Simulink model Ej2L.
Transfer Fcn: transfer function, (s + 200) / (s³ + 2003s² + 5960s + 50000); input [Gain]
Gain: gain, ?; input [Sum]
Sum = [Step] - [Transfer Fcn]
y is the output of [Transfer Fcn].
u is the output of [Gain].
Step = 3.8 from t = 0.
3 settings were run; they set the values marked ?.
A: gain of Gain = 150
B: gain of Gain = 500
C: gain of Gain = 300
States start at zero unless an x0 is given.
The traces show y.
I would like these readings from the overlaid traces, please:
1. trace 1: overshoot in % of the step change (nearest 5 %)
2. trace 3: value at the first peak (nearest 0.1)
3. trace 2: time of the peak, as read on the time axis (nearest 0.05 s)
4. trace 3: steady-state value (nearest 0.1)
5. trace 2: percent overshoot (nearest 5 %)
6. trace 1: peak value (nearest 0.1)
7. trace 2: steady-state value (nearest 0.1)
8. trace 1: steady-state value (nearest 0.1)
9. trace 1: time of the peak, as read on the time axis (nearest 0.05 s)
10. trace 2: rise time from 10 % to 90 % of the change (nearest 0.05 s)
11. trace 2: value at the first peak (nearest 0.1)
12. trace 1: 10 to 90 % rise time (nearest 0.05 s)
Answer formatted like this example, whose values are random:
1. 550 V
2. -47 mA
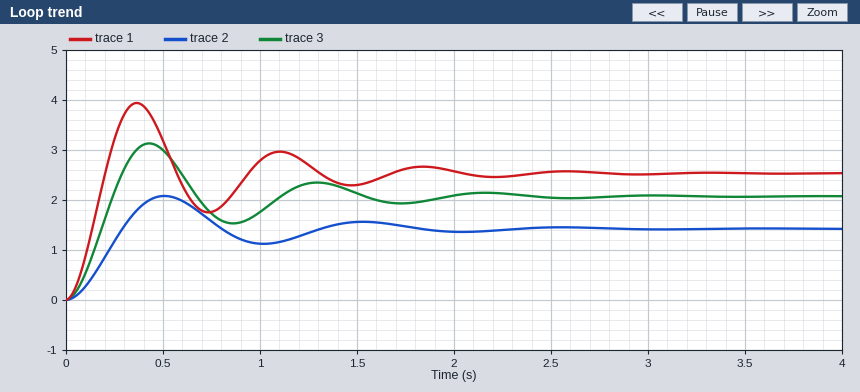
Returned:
1. 55 %
2. 3.1
3. 0.50 s
4. 2.1
5. 45 %
6. 3.9
7. 1.4
8. 2.5
9. 0.35 s
10. 0.20 s
11. 2.1
12. 0.15 s
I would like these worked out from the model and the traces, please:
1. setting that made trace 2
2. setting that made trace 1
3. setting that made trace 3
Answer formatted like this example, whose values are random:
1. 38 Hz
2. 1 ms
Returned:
1. A
2. B
3. C
